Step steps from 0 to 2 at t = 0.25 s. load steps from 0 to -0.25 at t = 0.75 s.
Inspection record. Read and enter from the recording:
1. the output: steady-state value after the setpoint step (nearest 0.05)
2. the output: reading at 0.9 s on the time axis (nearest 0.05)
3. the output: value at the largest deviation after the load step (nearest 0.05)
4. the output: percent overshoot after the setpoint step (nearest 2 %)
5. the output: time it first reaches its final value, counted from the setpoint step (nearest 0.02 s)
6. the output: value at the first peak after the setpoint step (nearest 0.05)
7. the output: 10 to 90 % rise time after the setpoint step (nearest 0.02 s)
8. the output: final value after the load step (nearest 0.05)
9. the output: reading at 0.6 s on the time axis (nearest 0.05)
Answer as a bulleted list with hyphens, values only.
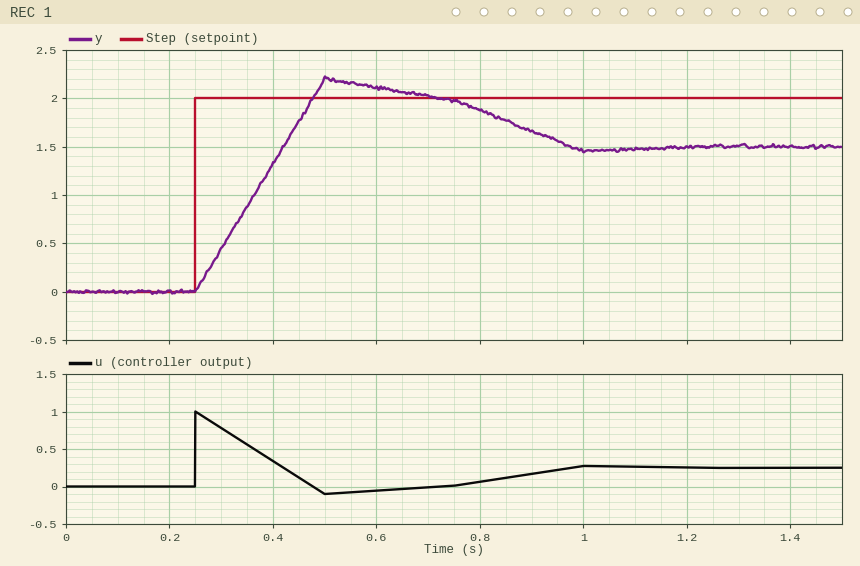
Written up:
- 2.00
- 1.65
- 1.45
- 10 %
- 0.22 s
- 2.20
- 0.18 s
- 1.50
- 2.10
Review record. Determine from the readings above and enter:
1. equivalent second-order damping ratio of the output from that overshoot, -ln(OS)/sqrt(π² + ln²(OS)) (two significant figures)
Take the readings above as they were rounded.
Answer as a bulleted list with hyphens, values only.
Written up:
- 0.59
